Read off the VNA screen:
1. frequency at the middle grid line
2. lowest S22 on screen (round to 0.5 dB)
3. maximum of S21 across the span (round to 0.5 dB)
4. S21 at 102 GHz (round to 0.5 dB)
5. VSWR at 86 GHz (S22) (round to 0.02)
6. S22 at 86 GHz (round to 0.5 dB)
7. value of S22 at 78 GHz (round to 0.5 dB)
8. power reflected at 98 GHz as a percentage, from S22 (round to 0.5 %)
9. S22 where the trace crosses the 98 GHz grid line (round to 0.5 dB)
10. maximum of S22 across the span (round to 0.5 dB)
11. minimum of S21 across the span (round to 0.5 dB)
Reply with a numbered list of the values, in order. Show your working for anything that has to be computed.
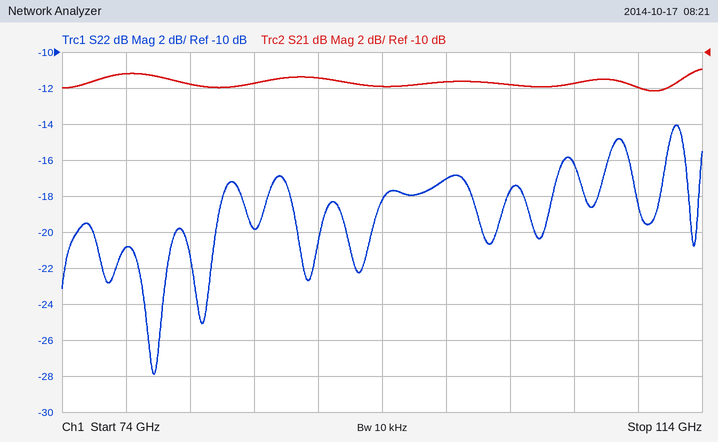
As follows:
1. 94 GHz
2. -28.0 dB
3. -11.0 dB
4. -12.0 dB
5. |Γ| = 10^(-20/20) = 0.1000; VSWR = (1 + 0.1000)/(1 − 0.1000) ≈ 1.22
6. -20.0 dB
7. -21.0 dB
8. 10^(-17/10) ≈ 2.0 %
9. -17.0 dB
10. -14.0 dB
11. -12.0 dB
